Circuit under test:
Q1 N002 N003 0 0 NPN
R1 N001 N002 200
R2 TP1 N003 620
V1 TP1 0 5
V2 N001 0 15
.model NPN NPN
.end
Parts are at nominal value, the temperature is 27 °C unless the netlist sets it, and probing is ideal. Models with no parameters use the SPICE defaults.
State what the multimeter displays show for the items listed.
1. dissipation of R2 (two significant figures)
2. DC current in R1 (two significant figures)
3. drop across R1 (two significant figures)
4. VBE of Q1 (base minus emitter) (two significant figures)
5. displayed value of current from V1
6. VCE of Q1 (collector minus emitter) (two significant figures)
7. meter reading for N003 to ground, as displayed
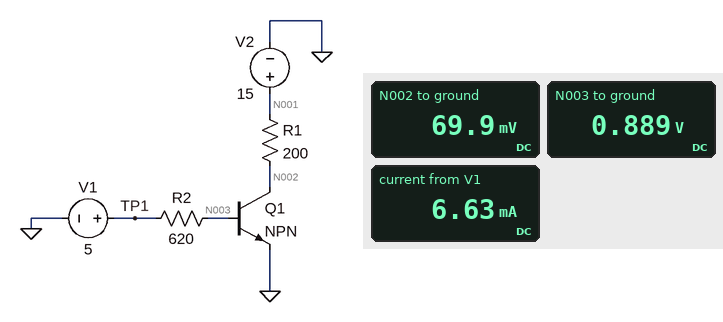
27 mW
75 mA
15 V
890 mV
6.63 mA
70 mV
0.889 V
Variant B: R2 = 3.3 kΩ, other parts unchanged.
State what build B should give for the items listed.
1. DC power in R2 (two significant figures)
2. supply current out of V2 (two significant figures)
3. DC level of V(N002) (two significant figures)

5.1 mW
74 mA
130 mV
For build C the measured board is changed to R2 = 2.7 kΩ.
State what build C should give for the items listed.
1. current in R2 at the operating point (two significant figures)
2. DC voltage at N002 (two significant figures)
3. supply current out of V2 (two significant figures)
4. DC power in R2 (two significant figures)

1.5 mA
120 mV
74 mA
6.3 mW
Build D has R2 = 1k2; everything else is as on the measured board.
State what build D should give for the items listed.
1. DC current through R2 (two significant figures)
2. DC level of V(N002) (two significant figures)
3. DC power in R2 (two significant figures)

3.4 mA
88 mV
14 mW
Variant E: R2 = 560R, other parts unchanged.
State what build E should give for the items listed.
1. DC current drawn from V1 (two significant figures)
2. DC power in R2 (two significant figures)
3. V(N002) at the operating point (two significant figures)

7.3 mA
30 mW
67 mV
